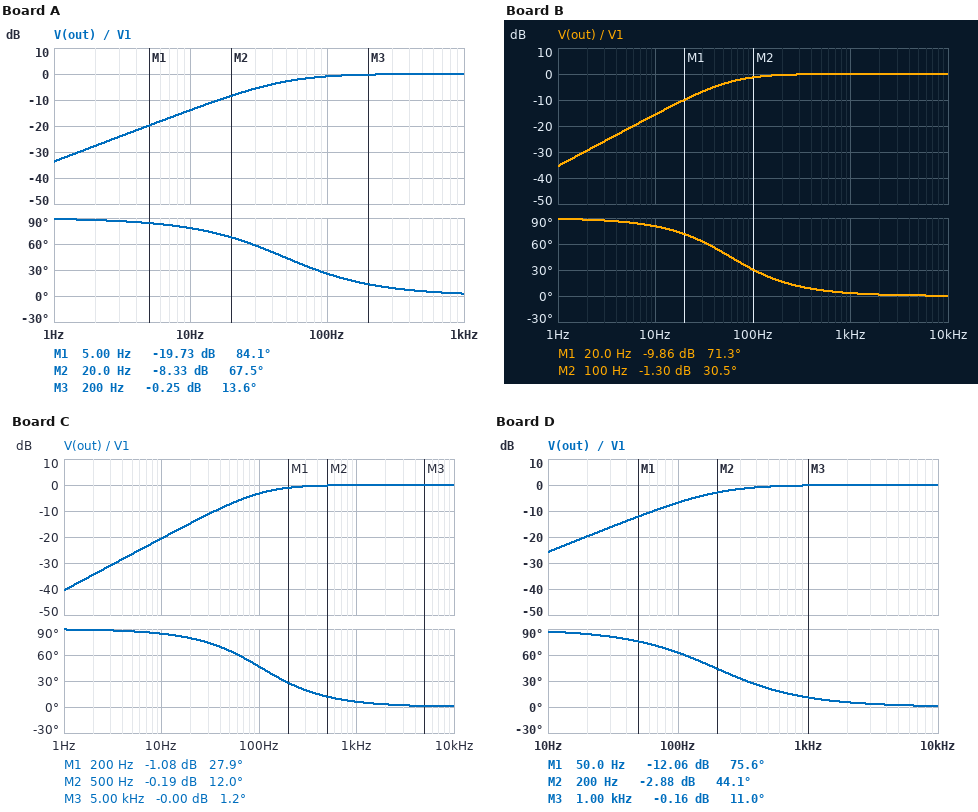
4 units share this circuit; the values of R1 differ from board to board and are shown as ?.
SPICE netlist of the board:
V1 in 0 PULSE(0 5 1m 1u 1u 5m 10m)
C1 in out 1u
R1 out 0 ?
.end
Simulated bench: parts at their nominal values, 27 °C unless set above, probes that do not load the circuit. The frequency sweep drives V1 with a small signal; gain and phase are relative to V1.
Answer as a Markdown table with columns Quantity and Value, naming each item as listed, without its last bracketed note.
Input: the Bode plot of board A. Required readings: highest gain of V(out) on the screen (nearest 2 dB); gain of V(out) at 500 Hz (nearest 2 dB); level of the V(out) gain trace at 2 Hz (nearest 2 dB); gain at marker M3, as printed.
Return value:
| Quantity | Value |
|---|---|
| highest gain of V(out) on the screen | 0 dB |
| gain of V(out) at 500 Hz | 0 dB |
| level of the V(out) gain trace at 2 Hz | -28 dB |
| gain at marker M3, as printed | -0.25 dB |
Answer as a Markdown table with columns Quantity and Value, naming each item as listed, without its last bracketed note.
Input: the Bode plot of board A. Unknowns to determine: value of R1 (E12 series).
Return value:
| Quantity | Value |
|---|---|
| value of R1 | 3.3 kΩ |
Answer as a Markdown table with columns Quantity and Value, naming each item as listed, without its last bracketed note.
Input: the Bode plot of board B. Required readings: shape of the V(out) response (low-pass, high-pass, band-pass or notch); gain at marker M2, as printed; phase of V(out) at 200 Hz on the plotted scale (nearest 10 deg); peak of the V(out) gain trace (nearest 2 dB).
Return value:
| Quantity | Value |
|---|---|
| shape of the V(out) response | high-pass |
| gain at marker M2, as printed | -1.30 dB |
| phase of V(out) at 200 Hz on the plotted scale | 20 deg |
| peak of the V(out) gain trace | 0 dB |
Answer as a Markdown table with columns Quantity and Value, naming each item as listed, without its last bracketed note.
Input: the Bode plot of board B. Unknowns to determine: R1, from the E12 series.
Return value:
| Quantity | Value |
|---|---|
| R1, from the E12 series | 2.7 kΩ |
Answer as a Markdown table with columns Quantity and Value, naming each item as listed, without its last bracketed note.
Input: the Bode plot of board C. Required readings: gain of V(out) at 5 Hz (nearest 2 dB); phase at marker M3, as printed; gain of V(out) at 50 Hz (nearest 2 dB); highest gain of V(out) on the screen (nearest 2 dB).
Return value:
| Quantity | Value |
|---|---|
| gain of V(out) at 5 Hz | -26 dB |
| phase at marker M3, as printed | 1.2 deg |
| gain of V(out) at 50 Hz | -8 dB |
| highest gain of V(out) on the screen | 0 dB |
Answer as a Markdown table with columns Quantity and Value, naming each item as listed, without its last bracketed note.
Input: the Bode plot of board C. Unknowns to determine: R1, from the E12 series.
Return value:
| Quantity | Value |
|---|---|
| R1, from the E12 series | 1.5 kΩ |
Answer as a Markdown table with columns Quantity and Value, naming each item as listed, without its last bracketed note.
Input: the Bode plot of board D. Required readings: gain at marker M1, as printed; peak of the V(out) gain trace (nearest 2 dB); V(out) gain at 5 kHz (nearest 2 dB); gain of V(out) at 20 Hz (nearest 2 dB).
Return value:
| Quantity | Value |
|---|---|
| gain at marker M1, as printed | -12.06 dB |
| peak of the V(out) gain trace | 0 dB |
| V(out) gain at 5 kHz | 0 dB |
| gain of V(out) at 20 Hz | -20 dB |
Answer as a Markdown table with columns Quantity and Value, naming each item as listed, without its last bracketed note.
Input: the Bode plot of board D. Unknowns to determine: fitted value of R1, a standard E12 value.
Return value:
| Quantity | Value |
|---|---|
| fitted value of R1, a standard E12 value | 820 Ω |
